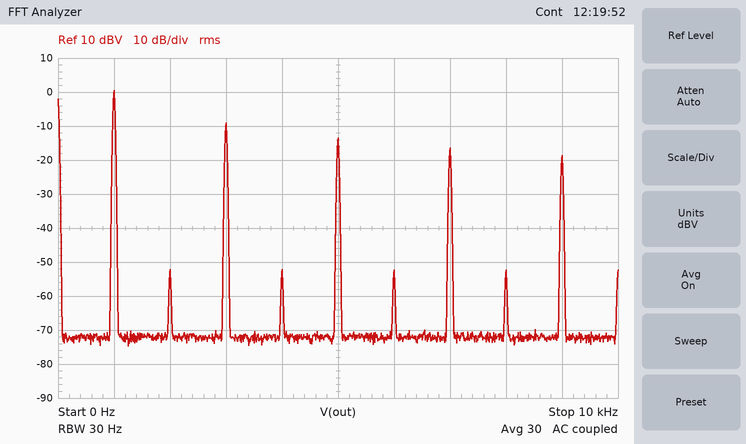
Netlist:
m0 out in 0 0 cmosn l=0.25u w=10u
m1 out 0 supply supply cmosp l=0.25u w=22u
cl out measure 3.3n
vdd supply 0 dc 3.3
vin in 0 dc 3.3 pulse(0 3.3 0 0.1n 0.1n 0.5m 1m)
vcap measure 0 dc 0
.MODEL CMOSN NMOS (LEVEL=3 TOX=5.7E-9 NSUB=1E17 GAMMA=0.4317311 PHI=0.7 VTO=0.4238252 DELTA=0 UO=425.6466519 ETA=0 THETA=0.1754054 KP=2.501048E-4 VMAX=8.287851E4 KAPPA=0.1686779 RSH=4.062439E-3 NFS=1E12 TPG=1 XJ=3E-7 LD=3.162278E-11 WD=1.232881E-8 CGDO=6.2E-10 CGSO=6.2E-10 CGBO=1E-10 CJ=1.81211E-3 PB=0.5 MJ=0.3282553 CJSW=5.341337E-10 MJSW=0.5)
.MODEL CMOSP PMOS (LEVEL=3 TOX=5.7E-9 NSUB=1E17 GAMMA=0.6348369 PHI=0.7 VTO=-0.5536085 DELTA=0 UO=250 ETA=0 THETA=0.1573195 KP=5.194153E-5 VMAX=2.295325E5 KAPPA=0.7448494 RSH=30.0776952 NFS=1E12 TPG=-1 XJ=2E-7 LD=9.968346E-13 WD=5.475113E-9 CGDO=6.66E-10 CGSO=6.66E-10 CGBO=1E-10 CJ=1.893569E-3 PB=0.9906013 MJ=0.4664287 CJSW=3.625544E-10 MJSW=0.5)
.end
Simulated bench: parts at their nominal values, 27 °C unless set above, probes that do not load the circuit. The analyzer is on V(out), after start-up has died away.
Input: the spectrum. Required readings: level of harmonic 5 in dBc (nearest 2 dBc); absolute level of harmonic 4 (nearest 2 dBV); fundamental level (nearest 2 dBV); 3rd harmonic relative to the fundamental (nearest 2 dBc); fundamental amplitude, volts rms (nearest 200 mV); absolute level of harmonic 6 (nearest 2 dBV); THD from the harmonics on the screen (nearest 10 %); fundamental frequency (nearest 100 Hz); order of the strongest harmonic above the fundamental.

-14 dBc
-52 dBV
0 dBV
-10 dBc
1.0 V
-52 dBV
40 %
1.0 kHz
3
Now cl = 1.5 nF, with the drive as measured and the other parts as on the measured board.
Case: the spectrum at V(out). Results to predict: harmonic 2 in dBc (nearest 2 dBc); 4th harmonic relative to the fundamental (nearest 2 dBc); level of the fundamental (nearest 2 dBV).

-60 dBc
-60 dBc
0 dBV
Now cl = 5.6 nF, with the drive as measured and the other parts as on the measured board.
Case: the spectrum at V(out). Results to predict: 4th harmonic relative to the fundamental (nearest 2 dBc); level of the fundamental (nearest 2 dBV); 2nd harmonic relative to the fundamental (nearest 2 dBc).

-48 dBc
0 dBV
-48 dBc
